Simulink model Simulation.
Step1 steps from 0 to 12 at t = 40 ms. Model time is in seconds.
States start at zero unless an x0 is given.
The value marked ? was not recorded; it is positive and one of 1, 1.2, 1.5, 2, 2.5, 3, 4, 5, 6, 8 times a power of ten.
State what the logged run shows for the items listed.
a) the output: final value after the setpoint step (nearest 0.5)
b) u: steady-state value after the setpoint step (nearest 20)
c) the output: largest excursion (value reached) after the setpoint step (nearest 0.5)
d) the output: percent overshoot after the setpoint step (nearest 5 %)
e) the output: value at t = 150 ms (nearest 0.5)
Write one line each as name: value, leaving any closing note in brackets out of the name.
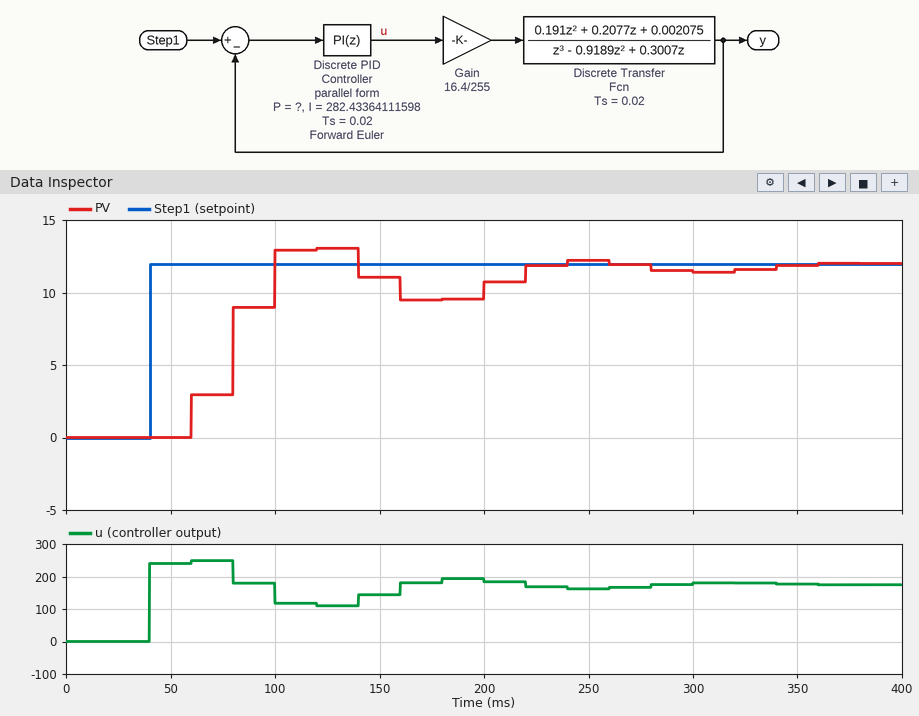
the output: final value after the setpoint step: 12.0
u: steady-state value after the setpoint step: 180
the output: largest excursion (value reached) after the setpoint step: 13.0
the output: percent overshoot after the setpoint step: 10 %
the output: value at t = 150 ms: 11.0
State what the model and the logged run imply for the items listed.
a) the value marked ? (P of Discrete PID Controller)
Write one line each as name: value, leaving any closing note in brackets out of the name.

the value marked ?: 20
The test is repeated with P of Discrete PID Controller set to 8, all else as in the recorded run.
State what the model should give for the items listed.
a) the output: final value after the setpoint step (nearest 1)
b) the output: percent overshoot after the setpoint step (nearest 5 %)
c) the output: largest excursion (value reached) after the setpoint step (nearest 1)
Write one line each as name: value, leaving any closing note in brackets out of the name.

the output: final value after the setpoint step: 12
the output: percent overshoot after the setpoint step: 15 %
the output: largest excursion (value reached) after the setpoint step: 14
